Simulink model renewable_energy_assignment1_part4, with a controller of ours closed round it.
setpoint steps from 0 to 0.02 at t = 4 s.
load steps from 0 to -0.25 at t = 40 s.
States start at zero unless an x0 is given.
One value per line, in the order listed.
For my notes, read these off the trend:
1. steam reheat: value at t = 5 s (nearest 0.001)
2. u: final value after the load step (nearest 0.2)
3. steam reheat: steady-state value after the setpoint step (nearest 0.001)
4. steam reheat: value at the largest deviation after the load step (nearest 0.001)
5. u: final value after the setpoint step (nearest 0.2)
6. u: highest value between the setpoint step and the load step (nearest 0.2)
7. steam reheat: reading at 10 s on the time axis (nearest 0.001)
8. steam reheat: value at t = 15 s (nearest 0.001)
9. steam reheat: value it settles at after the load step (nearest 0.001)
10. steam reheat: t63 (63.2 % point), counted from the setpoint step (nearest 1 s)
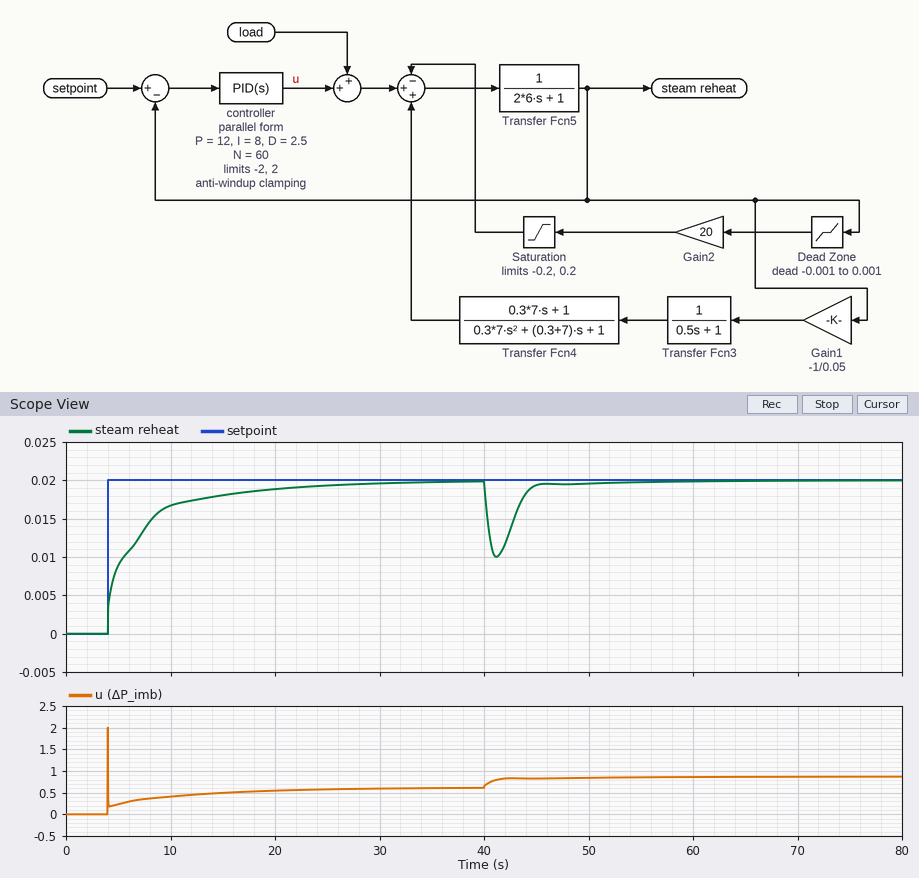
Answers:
0.009
0.8
0.020
0.010
0.6
2.0
0.017
0.018
0.020
3 s
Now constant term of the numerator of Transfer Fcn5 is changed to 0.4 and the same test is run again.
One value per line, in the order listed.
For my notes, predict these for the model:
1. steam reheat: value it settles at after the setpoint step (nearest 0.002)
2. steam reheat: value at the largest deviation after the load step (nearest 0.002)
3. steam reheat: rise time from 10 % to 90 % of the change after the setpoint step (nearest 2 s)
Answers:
0.020
0.012
8 s
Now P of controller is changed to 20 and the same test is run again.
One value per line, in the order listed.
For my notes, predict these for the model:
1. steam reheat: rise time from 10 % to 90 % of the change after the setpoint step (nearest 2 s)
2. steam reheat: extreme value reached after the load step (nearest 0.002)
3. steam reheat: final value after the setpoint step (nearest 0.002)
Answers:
12 s
0.012
0.020
